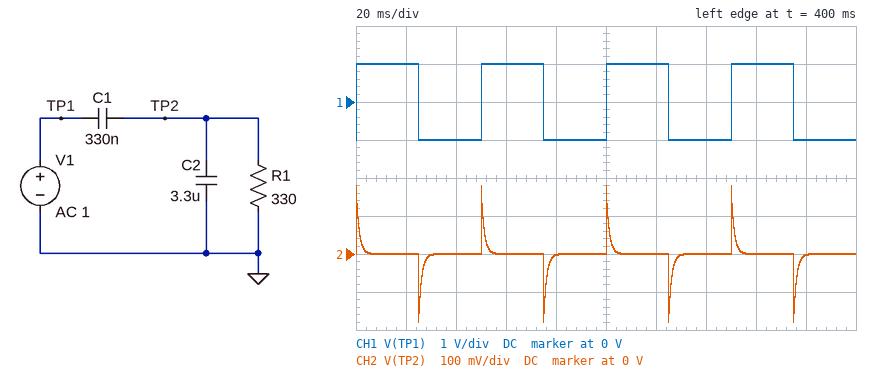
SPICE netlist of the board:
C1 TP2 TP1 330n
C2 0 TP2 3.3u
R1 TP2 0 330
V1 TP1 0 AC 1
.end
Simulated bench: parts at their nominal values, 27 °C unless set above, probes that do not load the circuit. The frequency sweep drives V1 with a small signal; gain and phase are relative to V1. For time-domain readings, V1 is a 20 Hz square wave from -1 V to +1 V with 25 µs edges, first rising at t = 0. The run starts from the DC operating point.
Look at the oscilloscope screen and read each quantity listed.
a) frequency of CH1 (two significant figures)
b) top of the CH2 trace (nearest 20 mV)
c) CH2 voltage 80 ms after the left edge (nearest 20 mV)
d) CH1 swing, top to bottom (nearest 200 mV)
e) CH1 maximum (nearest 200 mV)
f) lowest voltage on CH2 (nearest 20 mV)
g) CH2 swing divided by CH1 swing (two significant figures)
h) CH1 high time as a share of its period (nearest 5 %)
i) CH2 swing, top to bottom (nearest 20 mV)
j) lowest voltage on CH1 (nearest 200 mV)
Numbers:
20 Hz
180 mV
0 V
2.0 V
1.0 V
-180 mV
0.18
50 %
360 mV
-1.0 V
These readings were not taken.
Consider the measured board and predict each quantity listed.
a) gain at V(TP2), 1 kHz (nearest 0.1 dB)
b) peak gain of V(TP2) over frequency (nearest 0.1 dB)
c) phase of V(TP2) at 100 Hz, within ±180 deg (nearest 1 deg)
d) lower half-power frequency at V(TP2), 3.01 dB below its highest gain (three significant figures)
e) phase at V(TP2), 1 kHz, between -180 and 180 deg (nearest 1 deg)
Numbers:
-20.9 dB
-20.8 dB
53 deg
133 Hz
8 deg
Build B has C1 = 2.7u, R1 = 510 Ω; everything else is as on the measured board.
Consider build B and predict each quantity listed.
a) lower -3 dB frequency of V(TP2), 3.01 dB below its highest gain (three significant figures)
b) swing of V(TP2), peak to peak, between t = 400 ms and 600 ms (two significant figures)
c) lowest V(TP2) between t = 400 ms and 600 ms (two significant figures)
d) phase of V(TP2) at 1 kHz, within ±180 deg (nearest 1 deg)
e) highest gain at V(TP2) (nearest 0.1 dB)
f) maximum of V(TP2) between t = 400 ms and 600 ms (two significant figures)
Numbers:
52.0 Hz
1.8 V
-900 mV
3 deg
-6.9 dB
900 mV
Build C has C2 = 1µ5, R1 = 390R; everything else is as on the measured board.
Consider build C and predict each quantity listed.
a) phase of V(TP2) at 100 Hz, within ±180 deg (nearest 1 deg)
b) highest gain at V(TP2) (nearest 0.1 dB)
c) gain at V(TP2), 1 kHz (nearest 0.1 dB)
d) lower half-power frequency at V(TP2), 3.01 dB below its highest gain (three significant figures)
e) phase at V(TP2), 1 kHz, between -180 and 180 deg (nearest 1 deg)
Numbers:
66 deg
-14.9 dB
-15.1 dB
223 Hz
13 deg
